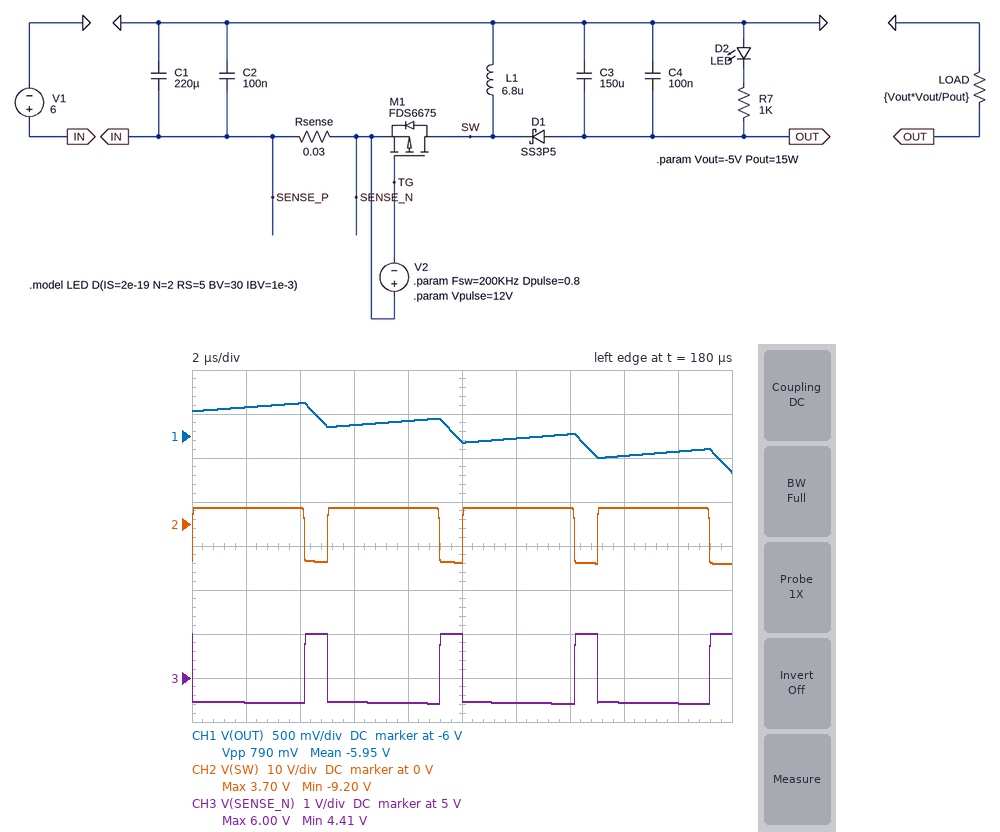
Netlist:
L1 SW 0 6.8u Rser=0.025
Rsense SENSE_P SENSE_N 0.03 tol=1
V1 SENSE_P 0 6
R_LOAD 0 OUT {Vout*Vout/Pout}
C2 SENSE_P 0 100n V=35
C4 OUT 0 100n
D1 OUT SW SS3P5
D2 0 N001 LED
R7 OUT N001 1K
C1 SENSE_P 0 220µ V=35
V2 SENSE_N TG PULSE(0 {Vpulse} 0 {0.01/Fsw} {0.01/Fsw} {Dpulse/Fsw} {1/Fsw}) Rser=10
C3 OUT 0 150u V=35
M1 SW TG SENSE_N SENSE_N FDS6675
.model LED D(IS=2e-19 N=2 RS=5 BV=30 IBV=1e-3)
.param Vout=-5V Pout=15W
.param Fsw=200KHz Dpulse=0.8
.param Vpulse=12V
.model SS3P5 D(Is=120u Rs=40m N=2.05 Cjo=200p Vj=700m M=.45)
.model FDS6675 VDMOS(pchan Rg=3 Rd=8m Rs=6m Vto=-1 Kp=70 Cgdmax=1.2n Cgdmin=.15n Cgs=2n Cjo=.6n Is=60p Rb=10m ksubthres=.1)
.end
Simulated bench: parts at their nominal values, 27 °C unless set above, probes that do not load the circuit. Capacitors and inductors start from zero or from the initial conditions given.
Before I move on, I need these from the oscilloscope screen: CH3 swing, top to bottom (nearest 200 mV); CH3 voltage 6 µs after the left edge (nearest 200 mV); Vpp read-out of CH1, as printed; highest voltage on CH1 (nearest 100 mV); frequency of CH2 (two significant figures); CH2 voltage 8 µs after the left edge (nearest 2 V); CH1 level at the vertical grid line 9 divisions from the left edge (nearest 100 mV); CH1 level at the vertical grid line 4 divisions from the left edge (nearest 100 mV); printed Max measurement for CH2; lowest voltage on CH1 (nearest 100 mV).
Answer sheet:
1.6 V
4.4 V
790 mV
-5.6 V
200 kHz
4 V
-6.2 V
-5.8 V
3.70 V
-6.4 V
